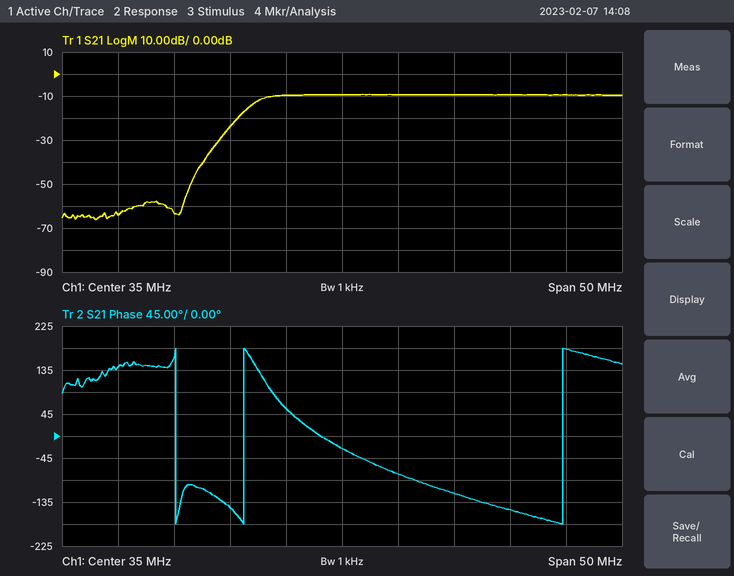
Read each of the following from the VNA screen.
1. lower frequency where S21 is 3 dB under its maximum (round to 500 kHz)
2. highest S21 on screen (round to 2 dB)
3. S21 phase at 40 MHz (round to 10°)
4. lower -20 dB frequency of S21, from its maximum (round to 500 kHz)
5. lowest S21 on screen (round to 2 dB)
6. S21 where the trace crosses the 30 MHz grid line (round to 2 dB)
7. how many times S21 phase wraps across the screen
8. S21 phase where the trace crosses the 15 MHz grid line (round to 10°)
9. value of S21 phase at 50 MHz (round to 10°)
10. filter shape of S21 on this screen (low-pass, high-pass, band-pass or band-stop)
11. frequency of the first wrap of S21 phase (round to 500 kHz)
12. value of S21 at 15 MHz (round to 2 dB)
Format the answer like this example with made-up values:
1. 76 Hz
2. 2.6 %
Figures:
1. 27.5 MHz
2. -10 dB
3. -80°
4. 24.0 MHz
5. -66 dB
6. -10 dB
7. 3
8. 140°
9. -150°
10. high-pass
11. 20.0 MHz
12. -64 dB
